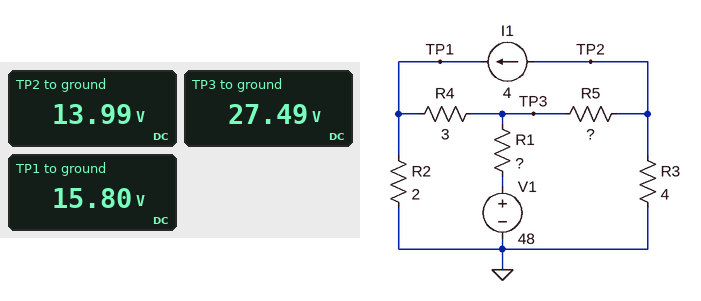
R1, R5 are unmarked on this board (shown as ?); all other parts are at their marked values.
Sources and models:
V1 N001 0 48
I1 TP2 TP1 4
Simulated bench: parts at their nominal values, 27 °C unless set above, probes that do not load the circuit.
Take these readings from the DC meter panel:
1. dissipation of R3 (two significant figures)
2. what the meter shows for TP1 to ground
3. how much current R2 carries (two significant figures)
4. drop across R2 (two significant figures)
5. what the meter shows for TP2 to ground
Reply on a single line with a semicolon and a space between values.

49 W; 15.80 V; 7.9 A; 16 V; 13.99 V
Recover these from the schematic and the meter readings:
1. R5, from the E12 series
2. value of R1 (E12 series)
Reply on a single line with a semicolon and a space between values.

1.8 Ω; 1.8 Ω
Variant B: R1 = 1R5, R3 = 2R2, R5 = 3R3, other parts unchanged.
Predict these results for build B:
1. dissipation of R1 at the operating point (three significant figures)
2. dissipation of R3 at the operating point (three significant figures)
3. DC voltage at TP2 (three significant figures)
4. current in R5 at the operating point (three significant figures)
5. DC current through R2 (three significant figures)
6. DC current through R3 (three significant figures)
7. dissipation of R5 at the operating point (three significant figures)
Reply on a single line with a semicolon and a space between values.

204 W; 21.8 W; 6.93 V; 7.15 A; 8.50 A; 3.15 A; 169 W
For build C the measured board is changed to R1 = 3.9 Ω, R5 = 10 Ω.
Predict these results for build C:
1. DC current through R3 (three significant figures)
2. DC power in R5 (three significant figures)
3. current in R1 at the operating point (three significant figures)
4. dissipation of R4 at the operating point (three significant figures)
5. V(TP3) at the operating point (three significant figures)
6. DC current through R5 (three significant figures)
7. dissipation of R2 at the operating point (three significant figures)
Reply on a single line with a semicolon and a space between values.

1.13 A; 82.4 W; 6.11 A; 31.4 W; 24.2 V; 2.87 A; 105 W
